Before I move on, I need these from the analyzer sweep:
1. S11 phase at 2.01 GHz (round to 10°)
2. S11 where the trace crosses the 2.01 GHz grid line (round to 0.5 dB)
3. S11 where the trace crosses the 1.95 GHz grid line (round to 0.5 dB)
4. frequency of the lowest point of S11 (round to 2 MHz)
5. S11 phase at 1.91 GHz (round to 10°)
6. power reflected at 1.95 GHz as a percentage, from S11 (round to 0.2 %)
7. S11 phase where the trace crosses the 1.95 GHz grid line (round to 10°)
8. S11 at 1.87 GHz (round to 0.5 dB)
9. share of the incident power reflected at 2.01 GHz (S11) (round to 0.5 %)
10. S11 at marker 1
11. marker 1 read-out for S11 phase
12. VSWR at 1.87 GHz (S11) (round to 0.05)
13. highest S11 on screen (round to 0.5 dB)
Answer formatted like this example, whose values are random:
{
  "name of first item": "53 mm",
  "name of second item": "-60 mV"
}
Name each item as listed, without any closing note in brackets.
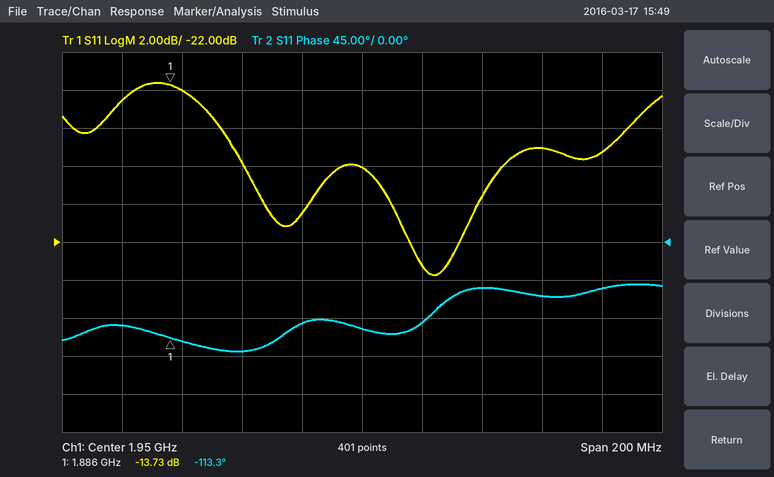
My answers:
{
  "S11 phase at 2.01 GHz": "-60°",
  "S11 where the trace crosses the 2.01 GHz grid line": "-17.0 dB",
  "S11 where the trace crosses the 1.95 GHz grid line": "-18.0 dB",
  "frequency of the lowest point of S11": "1.974 GHz",
  "S11 phase at 1.91 GHz": "-130°",
  "power reflected at 1.95 GHz as a percentage, from S11": "1.6 %",
  "S11 phase where the trace crosses the 1.95 GHz grid line": "-100°",
  "S11 at 1.87 GHz": "-14.5 dB",
  "share of the incident power reflected at 2.01 GHz (S11)": "2.0 %",
  "S11 at marker 1": "-13.73 dB",
  "marker 1 read-out for S11 phase": "-113.3°",
  "VSWR at 1.87 GHz (S11)": "1.45",
  "highest S11 on screen": "-13.5 dB"
}
